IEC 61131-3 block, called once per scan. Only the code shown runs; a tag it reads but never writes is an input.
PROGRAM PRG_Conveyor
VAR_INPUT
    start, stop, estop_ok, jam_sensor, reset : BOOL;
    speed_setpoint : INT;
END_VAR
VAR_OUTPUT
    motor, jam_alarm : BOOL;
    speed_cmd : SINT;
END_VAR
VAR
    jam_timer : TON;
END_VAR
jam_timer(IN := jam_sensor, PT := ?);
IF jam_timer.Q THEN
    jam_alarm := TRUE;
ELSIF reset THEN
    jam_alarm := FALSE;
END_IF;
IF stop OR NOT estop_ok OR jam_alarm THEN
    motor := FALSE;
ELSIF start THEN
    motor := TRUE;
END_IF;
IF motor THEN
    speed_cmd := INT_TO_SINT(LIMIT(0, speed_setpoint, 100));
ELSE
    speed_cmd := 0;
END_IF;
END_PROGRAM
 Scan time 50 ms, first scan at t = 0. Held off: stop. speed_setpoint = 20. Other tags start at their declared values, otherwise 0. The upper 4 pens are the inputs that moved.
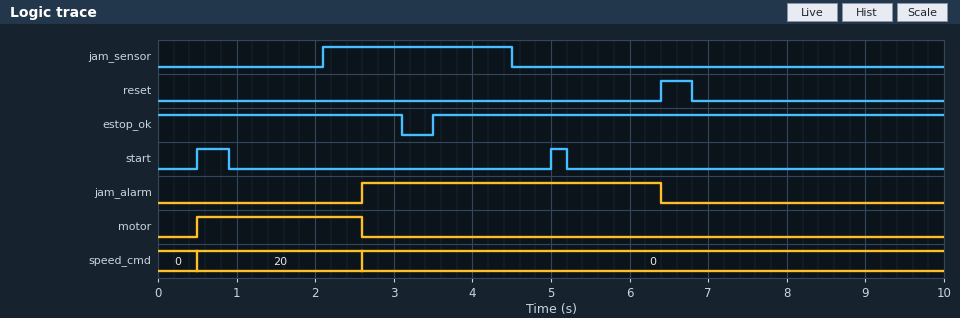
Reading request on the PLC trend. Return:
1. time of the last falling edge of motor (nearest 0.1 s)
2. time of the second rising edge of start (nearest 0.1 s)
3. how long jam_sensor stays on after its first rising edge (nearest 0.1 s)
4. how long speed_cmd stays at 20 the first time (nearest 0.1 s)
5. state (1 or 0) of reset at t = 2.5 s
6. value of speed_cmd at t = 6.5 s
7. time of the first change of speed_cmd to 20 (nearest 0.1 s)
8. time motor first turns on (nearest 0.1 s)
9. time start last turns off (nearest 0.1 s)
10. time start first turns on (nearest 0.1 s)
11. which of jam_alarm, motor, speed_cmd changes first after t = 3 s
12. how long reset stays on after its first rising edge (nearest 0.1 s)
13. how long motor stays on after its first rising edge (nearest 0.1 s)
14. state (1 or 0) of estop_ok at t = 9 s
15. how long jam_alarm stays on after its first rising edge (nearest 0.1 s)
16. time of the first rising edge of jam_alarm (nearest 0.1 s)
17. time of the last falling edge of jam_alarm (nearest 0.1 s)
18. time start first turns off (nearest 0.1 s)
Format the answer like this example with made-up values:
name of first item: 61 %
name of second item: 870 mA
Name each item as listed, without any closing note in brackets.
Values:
time of the last falling edge of motor: 2.6 s
time of the second rising edge of start: 5.0 s
how long jam_sensor stays on after its first rising edge: 2.4 s
how long speed_cmd stays at 20 the first time: 2.1 s
state (1 or 0) of reset at t = 2.5 s: 0
value of speed_cmd at t = 6.5 s: 0
time of the first change of speed_cmd to 20: 0.5 s
time motor first turns on: 0.5 s
time start last turns off: 5.2 s
time start first turns on: 0.5 s
which of jam_alarm, motor, speed_cmd changes first after t = 3 s: jam_alarm
how long reset stays on after its first rising edge: 0.4 s
how long motor stays on after its first rising edge: 2.1 s
state (1 or 0) of estop_ok at t = 9 s: 1
how long jam_alarm stays on after its first rising edge: 3.8 s
time of the first rising edge of jam_alarm: 2.6 s
time of the last falling edge of jam_alarm: 6.4 s
time start first turns off: 0.9 s
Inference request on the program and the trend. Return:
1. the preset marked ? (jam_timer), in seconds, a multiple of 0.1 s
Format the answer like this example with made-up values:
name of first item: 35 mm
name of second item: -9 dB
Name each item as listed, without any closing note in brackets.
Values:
the preset marked ? (jam_timer), in seconds, a multiple of 0.1 s: 0.5 s
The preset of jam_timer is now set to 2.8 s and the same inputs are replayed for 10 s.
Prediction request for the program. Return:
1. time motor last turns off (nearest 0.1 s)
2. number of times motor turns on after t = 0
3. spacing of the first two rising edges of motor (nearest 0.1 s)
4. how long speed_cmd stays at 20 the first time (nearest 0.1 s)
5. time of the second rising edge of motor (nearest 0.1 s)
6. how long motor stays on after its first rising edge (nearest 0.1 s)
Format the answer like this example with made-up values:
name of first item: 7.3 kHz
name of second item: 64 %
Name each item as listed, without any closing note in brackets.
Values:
time motor last turns off: 3.1 s
number of times motor turns on after t = 0: 2
spacing of the first two rising edges of motor: 4.5 s
how long speed_cmd stays at 20 the first time: 2.6 s
time of the second rising edge of motor: 5.0 s
how long motor stays on after its first rising edge: 2.6 s
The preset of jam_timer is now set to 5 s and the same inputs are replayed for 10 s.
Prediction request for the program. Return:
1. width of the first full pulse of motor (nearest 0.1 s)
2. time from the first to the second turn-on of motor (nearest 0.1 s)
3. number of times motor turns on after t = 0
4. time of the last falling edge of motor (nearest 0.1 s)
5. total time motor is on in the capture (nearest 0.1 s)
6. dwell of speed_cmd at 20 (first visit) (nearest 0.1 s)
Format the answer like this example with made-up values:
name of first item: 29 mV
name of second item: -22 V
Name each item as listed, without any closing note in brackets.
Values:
width of the first full pulse of motor: 2.6 s
time from the first to the second turn-on of motor: 4.5 s
number of times motor turns on after t = 0: 2
time of the last falling edge of motor: 3.1 s
total time motor is on in the capture: 7.6 s
dwell of speed_cmd at 20 (first visit): 2.6 s
